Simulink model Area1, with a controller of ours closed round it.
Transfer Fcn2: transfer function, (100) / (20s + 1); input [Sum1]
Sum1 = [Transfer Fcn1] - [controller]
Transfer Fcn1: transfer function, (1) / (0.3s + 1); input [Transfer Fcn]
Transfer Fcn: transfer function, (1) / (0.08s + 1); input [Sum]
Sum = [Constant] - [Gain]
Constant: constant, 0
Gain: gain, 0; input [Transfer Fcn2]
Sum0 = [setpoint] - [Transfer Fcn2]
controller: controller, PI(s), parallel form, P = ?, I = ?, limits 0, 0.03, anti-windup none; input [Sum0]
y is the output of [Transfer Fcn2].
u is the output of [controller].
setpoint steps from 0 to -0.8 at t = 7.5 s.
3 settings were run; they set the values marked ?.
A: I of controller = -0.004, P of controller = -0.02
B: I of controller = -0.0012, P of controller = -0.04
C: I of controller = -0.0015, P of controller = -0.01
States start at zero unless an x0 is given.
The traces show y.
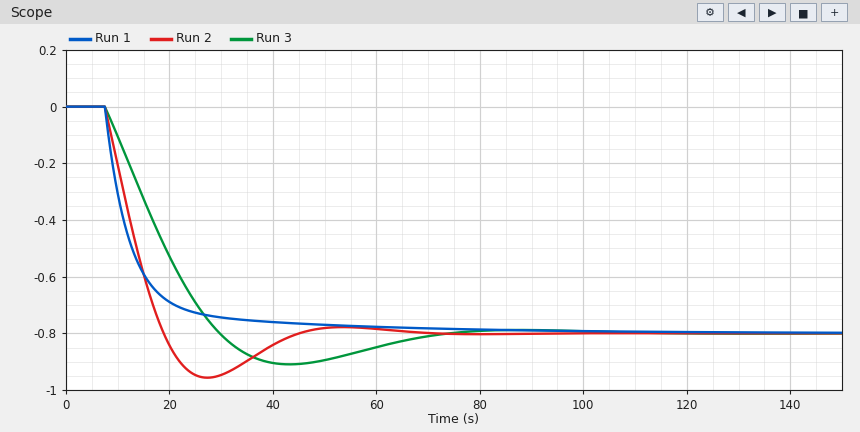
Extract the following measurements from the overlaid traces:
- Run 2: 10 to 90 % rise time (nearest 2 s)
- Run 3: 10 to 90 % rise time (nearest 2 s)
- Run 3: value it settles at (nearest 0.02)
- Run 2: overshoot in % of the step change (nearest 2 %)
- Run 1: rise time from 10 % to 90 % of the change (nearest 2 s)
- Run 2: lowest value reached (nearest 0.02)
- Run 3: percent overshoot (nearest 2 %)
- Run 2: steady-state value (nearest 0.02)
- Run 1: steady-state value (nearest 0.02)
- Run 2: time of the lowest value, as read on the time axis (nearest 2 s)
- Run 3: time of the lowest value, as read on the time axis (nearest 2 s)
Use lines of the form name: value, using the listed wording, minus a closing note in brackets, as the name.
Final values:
Run 2: 10 to 90 % rise time: 8 s
Run 3: 10 to 90 % rise time: 16 s
Run 3: value it settles at: -0.80
Run 2: overshoot in % of the step change: 20 %
Run 1: rise time from 10 % to 90 % of the change: 16 s
Run 2: lowest value reached: -0.96
Run 3: percent overshoot: 14 %
Run 2: steady-state value: -0.80
Run 1: steady-state value: -0.80
Run 2: time of the lowest value, as read on the time axis: 28 s
Run 3: time of the lowest value, as read on the time axis: 44 s
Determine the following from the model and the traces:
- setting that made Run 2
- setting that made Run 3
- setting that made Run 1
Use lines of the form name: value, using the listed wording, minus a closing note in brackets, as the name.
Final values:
setting that made Run 2: A
setting that made Run 3: C
setting that made Run 1: B
